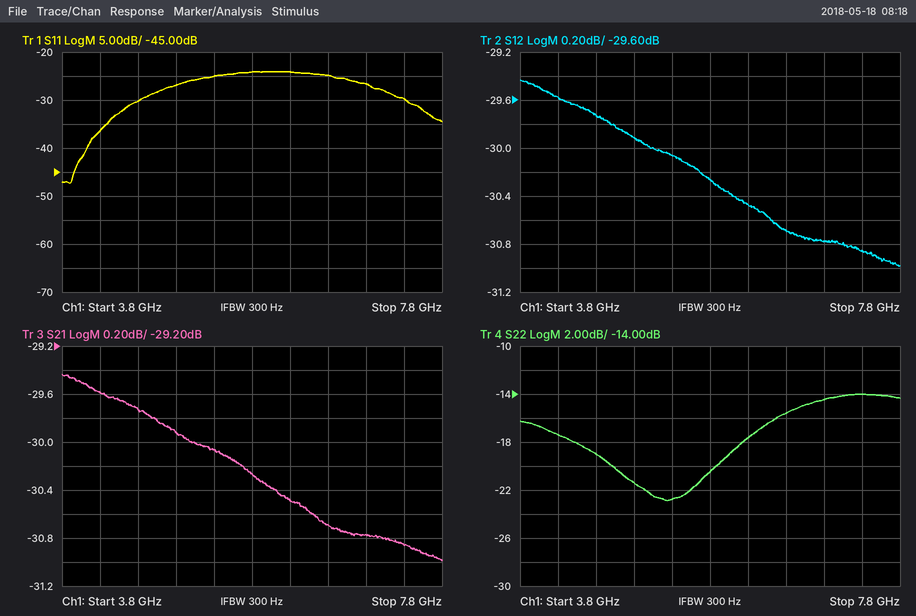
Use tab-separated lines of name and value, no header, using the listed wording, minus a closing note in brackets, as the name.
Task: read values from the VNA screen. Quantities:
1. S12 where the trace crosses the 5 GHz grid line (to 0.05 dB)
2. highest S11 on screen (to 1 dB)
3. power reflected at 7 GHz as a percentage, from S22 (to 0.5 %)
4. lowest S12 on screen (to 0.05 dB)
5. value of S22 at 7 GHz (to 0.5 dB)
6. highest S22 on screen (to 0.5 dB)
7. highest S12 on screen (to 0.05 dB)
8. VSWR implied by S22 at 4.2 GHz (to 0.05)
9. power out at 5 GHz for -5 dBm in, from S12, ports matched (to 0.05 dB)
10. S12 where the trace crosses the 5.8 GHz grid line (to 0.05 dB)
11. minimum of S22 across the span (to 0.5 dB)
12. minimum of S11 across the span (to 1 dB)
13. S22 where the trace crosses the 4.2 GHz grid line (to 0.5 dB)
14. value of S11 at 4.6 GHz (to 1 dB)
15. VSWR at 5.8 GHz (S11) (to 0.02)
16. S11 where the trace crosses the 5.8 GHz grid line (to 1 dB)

S12 where the trace crosses the 5 GHz grid line	-29.90 dB
highest S11 on screen	-24 dB
power reflected at 7 GHz as a percentage, from S22	3.5 %
lowest S12 on screen	-31.00 dB
value of S22 at 7 GHz	-14.5 dB
highest S22 on screen	-14.0 dB
highest S12 on screen	-29.45 dB
VSWR implied by S22 at 4.2 GHz	1.30
power out at 5 GHz for -5 dBm in, from S12, ports matched	-34.90 dBm
S12 where the trace crosses the 5.8 GHz grid line	-30.25 dB
minimum of S22 across the span	-23.0 dB
minimum of S11 across the span	-47 dB
S22 where the trace crosses the 4.2 GHz grid line	-17.5 dB
value of S11 at 4.6 GHz	-30 dB
VSWR at 5.8 GHz (S11)	1.14
S11 where the trace crosses the 5.8 GHz grid line	-24 dB
